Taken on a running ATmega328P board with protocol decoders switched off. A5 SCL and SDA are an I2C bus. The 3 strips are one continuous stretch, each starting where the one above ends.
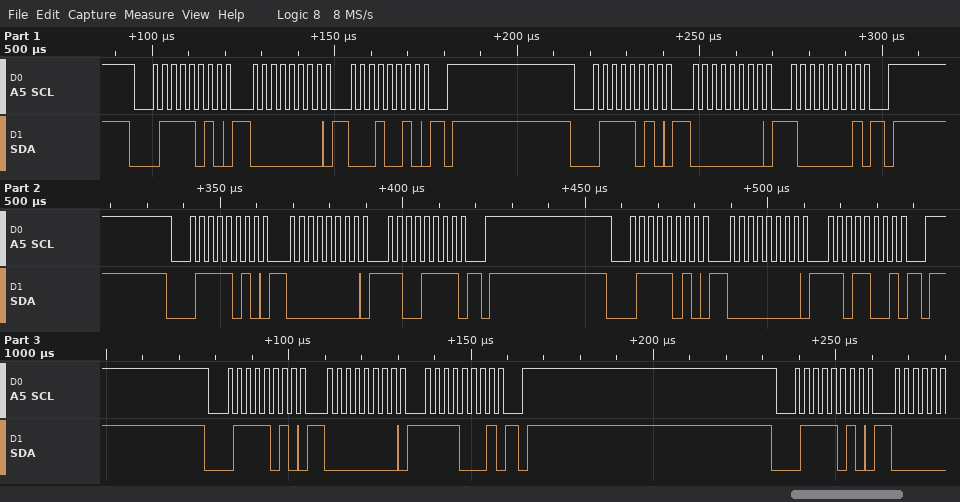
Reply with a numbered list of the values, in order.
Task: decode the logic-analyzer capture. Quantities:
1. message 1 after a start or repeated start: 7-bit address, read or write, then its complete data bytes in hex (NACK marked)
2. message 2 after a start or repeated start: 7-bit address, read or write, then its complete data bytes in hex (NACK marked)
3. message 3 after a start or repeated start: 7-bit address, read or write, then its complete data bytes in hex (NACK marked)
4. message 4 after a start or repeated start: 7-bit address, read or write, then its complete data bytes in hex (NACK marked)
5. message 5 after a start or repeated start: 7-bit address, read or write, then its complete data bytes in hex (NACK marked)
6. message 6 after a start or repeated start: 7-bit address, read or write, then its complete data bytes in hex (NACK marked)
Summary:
1. 0x3D write: 00 12
2. 0x3D write: 00 81
3. 0x3D write: 00 CF
4. 0x3D write: 00 D9
5. 0x3D write: 00 F1
6. 0x3D write
